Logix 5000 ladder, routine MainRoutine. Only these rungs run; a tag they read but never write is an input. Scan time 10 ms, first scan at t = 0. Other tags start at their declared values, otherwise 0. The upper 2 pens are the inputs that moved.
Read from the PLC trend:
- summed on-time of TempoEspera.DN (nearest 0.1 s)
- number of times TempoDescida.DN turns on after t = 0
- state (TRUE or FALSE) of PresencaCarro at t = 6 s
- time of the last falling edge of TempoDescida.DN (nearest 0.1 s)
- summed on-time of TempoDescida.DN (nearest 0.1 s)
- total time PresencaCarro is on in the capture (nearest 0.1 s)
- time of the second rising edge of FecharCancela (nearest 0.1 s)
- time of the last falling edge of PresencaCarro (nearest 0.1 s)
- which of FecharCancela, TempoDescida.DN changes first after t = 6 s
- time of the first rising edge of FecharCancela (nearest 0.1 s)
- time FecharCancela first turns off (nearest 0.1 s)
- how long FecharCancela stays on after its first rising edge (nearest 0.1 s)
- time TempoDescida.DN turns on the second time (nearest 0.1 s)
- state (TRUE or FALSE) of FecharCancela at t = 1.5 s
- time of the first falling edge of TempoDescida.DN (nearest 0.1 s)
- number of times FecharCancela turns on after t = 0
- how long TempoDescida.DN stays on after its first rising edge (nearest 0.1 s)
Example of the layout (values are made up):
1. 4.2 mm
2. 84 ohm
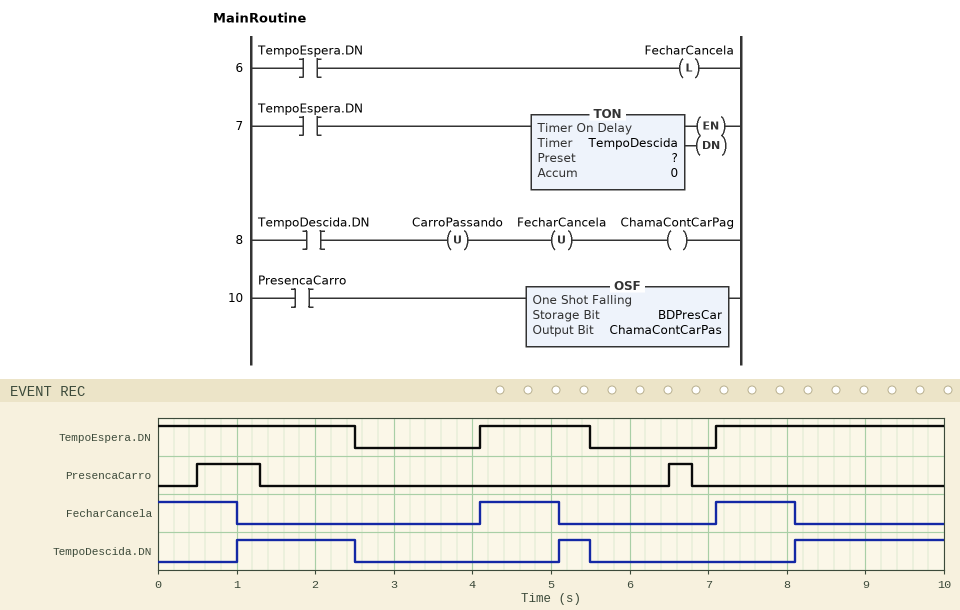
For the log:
1. 6.8 s
2. 3
3. FALSE
4. 5.5 s
5. 3.8 s
6. 1.1 s
7. 7.1 s
8. 6.8 s
9. FecharCancela
10. 4.1 s
11. 1.0 s
12. 1.0 s
13. 5.1 s
14. FALSE
15. 2.5 s
16. 2
17. 1.5 s
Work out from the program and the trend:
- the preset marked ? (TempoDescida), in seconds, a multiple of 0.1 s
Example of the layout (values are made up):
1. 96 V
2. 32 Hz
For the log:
1. 1.0 s
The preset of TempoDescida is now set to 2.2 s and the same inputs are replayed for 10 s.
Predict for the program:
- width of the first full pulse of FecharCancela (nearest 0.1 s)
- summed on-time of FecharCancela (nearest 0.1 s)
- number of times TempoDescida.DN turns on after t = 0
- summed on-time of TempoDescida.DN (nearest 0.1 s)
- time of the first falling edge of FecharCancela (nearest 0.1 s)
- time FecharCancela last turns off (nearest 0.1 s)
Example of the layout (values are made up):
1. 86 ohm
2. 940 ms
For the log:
1. 5.2 s
2. 7.4 s
3. 2
4. 1.0 s
5. 2.2 s
6. 9.3 s
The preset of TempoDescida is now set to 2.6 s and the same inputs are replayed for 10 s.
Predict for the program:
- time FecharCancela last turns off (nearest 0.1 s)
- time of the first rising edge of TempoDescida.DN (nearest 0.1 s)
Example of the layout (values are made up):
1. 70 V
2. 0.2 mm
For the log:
1. 9.7 s
2. 9.7 s
